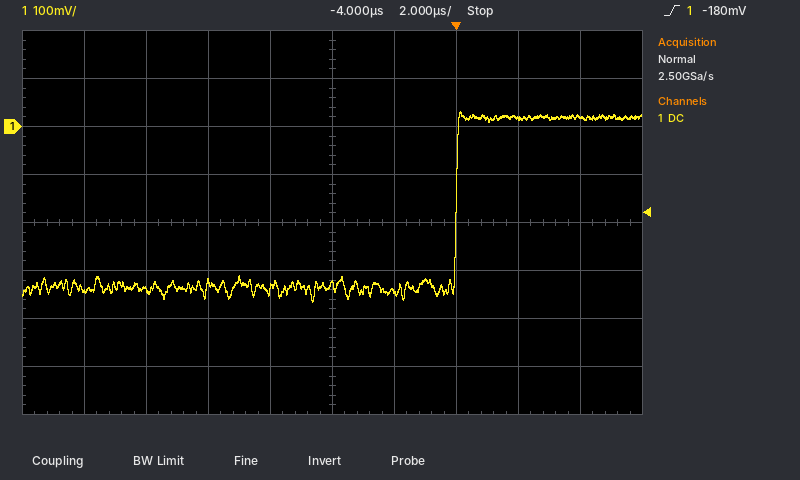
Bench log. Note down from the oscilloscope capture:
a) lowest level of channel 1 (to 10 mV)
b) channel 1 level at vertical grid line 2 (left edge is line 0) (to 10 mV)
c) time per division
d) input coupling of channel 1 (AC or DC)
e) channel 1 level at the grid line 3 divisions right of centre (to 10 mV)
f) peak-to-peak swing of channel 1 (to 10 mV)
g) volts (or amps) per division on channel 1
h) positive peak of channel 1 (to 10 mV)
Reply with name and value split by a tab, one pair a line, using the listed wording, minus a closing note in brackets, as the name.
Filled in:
lowest level of channel 1	-370 mV
channel 1 level at vertical grid line 2 (left edge is line 0)	-340 mV
time per division	2 µs
input coupling of channel 1	DC
channel 1 level at the grid line 3 divisions right of centre	20 mV
peak-to-peak swing of channel 1	400 mV
volts (or amps) per division on channel 1	100 mV
positive peak of channel 1	30 mV
